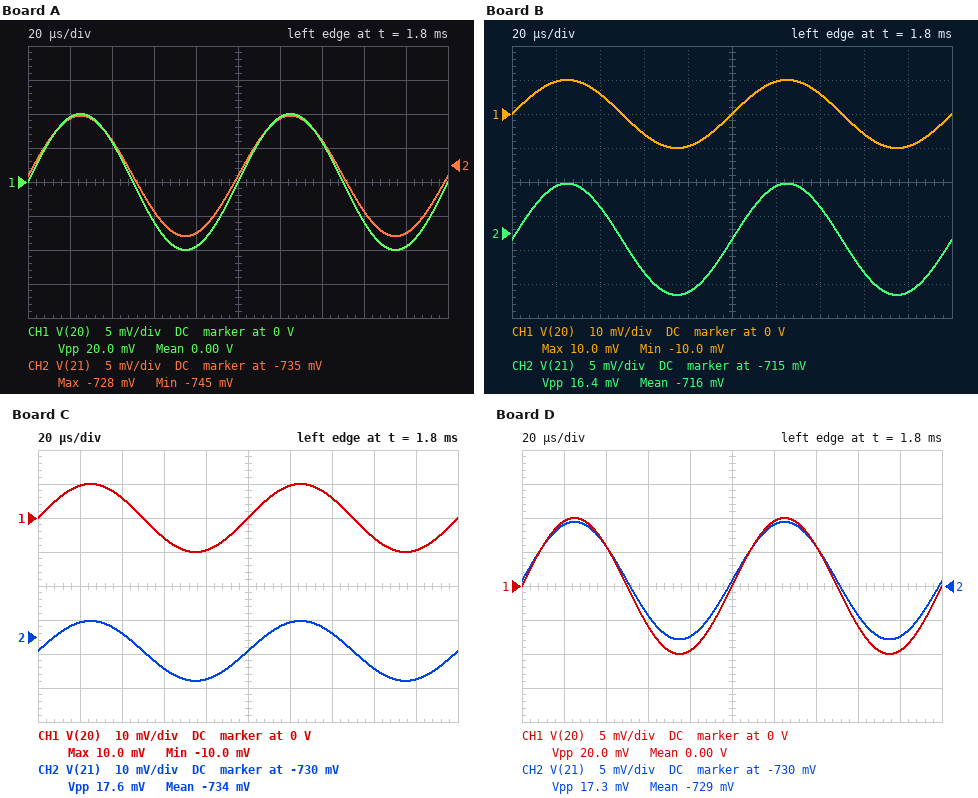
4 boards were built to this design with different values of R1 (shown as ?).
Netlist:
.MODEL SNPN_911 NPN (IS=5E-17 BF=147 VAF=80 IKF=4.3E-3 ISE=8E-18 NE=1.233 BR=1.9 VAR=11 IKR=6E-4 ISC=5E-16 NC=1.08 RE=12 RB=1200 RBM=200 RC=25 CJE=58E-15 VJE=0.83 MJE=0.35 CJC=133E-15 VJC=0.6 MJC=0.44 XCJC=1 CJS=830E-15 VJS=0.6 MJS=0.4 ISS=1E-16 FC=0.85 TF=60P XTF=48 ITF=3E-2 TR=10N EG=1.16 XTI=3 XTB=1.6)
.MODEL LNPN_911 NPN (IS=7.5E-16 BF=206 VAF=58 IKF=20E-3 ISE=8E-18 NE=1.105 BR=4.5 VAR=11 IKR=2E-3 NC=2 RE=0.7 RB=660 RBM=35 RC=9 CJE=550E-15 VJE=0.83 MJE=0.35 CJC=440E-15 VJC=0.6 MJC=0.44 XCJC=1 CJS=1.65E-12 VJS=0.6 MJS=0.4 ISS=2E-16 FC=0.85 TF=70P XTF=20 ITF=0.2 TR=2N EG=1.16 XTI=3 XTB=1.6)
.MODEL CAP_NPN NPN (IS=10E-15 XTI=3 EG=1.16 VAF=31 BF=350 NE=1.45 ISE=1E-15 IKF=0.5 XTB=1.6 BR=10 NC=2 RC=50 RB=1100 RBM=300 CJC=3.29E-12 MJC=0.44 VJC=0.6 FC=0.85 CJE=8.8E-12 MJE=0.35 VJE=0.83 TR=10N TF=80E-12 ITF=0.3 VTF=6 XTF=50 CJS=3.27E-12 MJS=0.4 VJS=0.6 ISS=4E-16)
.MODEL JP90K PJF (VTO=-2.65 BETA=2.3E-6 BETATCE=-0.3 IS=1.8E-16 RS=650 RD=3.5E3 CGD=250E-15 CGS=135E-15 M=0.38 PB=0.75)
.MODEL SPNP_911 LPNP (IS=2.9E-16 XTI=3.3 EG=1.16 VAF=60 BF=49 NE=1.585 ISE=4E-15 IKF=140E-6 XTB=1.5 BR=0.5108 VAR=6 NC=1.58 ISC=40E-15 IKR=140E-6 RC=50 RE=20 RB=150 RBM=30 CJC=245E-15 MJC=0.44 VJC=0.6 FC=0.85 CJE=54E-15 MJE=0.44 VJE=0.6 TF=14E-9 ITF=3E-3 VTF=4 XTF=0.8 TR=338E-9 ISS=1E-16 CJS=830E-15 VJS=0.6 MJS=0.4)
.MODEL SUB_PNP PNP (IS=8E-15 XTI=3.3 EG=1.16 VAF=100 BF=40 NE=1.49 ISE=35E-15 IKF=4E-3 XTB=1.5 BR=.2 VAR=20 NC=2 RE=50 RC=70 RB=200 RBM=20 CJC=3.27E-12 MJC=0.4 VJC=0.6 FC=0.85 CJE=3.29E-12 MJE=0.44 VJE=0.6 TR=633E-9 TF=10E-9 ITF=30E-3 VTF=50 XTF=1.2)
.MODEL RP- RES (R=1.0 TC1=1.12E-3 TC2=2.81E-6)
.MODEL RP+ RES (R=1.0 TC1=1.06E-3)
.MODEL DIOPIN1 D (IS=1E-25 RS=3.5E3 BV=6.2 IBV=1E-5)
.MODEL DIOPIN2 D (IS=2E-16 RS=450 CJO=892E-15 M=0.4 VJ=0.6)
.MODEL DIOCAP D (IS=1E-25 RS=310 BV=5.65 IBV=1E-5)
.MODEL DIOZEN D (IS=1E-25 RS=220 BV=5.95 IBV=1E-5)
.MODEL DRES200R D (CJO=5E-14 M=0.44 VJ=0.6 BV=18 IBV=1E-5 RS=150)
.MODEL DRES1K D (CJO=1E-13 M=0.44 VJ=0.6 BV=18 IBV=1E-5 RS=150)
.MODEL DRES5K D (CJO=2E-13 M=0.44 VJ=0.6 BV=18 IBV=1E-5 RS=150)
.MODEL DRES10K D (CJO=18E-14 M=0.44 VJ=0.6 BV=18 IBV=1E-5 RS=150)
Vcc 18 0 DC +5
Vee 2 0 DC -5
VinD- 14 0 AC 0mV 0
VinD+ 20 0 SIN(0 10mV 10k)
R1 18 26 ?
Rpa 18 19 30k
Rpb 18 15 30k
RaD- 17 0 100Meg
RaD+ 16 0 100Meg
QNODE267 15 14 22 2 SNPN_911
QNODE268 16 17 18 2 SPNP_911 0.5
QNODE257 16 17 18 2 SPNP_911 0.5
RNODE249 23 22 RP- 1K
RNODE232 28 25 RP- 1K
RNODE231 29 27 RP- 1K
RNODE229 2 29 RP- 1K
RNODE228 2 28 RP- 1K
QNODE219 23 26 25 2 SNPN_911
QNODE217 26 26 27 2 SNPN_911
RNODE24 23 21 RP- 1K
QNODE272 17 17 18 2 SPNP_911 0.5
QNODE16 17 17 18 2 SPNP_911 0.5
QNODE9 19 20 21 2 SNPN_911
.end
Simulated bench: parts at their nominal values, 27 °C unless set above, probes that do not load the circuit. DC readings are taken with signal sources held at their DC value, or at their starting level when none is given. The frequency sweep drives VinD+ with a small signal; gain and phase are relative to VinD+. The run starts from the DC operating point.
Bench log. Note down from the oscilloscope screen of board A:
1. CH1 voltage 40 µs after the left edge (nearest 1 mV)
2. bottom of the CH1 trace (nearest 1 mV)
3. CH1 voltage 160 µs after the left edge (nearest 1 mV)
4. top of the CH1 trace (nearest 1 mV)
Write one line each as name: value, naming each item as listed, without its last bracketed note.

CH1 voltage 40 µs after the left edge: 6 mV
bottom of the CH1 trace: -10 mV
CH1 voltage 160 µs after the left edge: -6 mV
top of the CH1 trace: 10 mV
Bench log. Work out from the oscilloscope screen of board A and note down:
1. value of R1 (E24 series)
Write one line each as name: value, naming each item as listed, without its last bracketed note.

value of R1: 43 kΩ
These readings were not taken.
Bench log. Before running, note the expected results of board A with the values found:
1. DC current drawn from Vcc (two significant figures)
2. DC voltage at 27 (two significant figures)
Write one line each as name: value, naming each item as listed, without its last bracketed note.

DC current drawn from Vcc: 410 µA
DC voltage at 27: -4.6 V
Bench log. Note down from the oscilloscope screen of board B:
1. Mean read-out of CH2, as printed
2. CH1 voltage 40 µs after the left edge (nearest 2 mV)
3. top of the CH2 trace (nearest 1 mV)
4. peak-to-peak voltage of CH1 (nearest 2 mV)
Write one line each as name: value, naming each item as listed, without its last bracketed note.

Mean read-out of CH2, as printed: -716 mV
CH1 voltage 40 µs after the left edge: 6 mV
top of the CH2 trace: -708 mV
peak-to-peak voltage of CH1: 20 mV
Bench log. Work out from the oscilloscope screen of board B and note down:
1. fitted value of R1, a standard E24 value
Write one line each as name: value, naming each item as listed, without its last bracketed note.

fitted value of R1, a standard E24 value: 91 kΩ
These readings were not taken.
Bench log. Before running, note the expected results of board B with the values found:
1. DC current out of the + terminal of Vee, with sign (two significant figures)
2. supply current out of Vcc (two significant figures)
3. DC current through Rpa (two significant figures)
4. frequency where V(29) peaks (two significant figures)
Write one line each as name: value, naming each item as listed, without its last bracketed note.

DC current out of the + terminal of Vee, with sign: -200 µA
supply current out of Vcc: 200 µA
DC current through Rpa: 49 µA
frequency where V(29) peaks: 190 MHz
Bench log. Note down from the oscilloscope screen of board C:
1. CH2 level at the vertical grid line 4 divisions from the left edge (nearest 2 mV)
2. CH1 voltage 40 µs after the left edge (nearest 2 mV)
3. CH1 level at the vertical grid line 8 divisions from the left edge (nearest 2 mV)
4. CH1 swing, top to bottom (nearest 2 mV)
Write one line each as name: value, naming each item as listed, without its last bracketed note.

CH2 level at the vertical grid line 4 divisions from the left edge: -742 mV
CH1 voltage 40 µs after the left edge: 6 mV
CH1 level at the vertical grid line 8 divisions from the left edge: -6 mV
CH1 swing, top to bottom: 20 mV
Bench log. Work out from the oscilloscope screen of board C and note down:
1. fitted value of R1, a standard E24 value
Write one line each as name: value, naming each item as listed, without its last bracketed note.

fitted value of R1, a standard E24 value: 47 kΩ
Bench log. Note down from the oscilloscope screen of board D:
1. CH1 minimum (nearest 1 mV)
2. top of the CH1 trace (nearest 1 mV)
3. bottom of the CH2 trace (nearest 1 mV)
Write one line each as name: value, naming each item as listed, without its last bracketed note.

CH1 minimum: -10 mV
top of the CH1 trace: 10 mV
bottom of the CH2 trace: -738 mV
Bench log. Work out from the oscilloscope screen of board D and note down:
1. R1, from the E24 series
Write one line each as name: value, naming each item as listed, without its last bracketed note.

R1, from the E24 series: 56 kΩ
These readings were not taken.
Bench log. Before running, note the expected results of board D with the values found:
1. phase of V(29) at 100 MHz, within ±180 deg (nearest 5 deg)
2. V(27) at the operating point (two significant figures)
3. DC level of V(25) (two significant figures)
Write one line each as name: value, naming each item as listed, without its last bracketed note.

phase of V(29) at 100 MHz, within ±180 deg: 30 deg
V(27) at the operating point: -4.7 V
DC level of V(25): -4.7 V
